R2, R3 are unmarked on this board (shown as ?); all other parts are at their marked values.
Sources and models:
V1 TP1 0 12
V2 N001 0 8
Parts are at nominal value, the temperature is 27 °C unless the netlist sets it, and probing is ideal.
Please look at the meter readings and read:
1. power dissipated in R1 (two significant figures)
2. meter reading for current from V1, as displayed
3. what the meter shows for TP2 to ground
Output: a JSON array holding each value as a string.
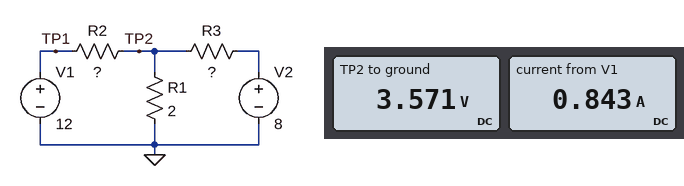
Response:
["6.4 W", "0.843 A", "3.571 V"]
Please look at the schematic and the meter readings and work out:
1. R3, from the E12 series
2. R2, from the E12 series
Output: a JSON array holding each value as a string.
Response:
["4.7 Ω", "10 Ω"]
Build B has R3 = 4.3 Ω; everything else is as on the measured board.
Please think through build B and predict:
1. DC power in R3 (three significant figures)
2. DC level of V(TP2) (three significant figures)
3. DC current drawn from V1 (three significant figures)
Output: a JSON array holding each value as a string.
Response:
["4.35 W", "3.68 V", "832 mA"]
